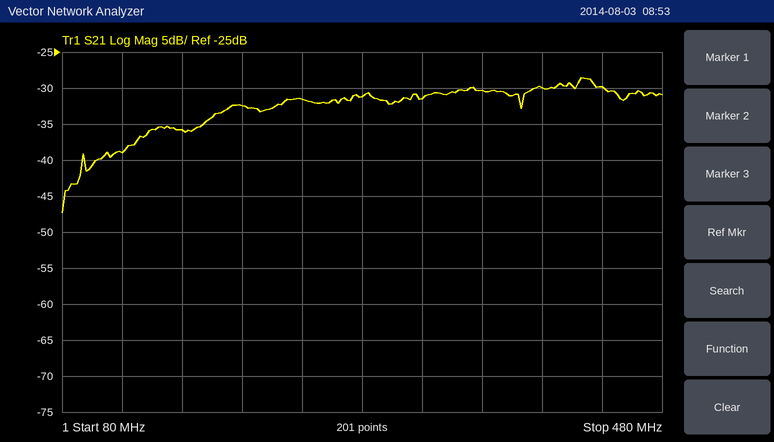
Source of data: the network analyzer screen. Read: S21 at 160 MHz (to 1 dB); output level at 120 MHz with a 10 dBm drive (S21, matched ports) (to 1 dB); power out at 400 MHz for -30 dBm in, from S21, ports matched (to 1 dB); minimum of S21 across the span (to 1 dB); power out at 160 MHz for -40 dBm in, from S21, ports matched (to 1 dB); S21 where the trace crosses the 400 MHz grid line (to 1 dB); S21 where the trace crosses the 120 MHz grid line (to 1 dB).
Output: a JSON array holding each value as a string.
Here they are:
["-36 dB", "-29 dBm", "-60 dBm", "-47 dB", "-76 dBm", "-30 dB", "-39 dB"]
